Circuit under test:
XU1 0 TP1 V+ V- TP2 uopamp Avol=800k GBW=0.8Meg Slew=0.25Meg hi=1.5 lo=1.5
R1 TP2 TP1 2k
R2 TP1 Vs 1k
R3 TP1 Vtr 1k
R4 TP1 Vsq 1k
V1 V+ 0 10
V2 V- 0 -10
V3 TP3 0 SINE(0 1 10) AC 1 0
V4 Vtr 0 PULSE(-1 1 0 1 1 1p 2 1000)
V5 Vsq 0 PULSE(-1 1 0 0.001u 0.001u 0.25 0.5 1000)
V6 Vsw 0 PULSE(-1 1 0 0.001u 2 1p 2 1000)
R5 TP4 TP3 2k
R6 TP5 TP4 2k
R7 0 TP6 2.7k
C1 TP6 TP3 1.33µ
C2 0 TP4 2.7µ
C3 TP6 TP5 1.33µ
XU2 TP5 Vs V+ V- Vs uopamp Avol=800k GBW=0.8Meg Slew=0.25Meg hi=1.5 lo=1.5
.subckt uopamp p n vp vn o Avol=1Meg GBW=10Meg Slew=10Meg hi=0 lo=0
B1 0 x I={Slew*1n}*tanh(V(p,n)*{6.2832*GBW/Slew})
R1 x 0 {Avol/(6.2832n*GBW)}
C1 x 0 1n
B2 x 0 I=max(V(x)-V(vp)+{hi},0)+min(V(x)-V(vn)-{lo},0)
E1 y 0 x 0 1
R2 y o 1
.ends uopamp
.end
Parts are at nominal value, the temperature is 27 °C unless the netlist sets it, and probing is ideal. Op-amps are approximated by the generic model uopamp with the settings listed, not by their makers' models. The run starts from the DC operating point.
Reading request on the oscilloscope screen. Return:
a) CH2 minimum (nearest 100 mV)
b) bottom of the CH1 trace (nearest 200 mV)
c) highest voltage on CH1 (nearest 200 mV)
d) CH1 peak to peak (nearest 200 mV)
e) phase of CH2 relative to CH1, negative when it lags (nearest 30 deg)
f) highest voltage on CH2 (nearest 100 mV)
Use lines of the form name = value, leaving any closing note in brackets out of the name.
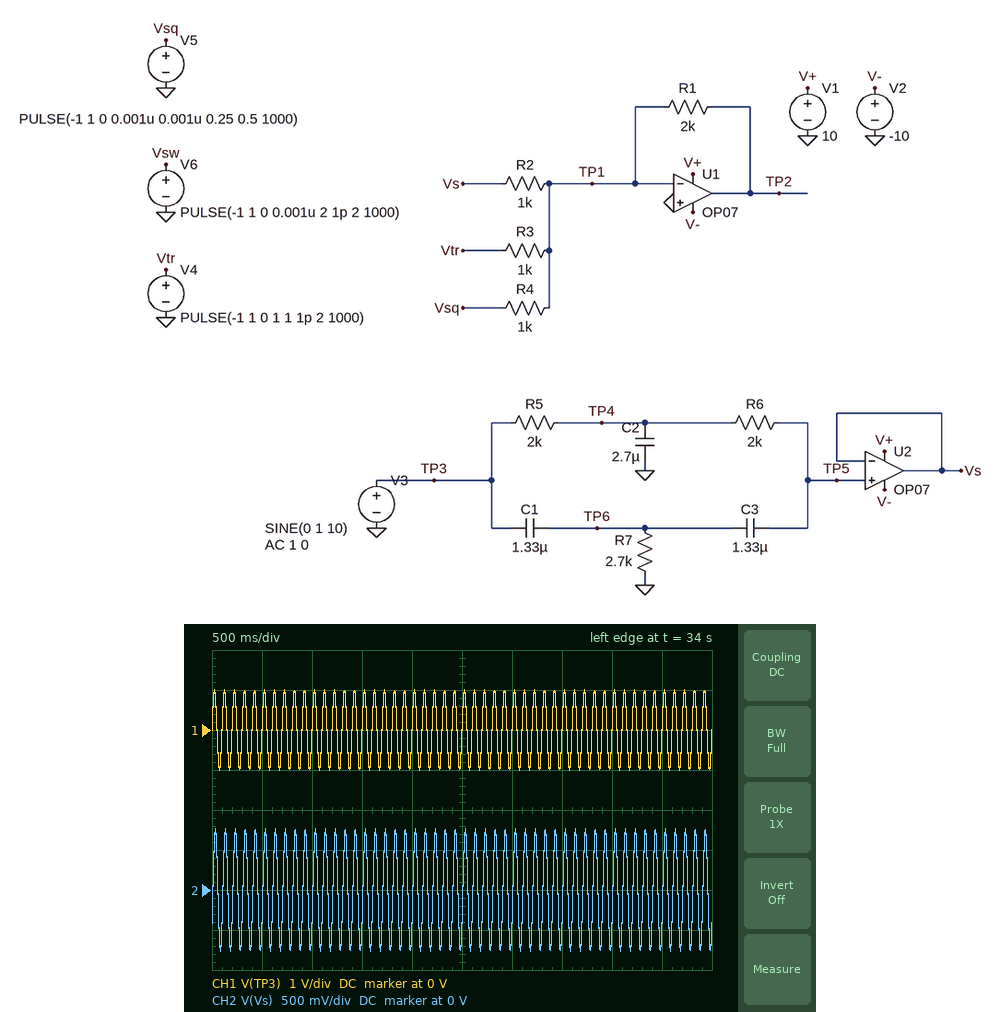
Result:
CH2 minimum = -800 mV
bottom of the CH1 trace = -1.0 V
highest voltage on CH1 = 1.0 V
CH1 peak to peak = 2.0 V
phase of CH2 relative to CH1, negative when it lags = -30 deg
highest voltage on CH2 = 800 mV
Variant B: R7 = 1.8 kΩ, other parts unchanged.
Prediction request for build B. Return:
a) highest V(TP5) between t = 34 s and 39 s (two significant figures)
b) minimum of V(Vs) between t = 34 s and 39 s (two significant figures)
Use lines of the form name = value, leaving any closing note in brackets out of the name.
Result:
highest V(TP5) between t = 34 s and 39 s = 790 mV
minimum of V(Vs) between t = 34 s and 39 s = -790 mV
